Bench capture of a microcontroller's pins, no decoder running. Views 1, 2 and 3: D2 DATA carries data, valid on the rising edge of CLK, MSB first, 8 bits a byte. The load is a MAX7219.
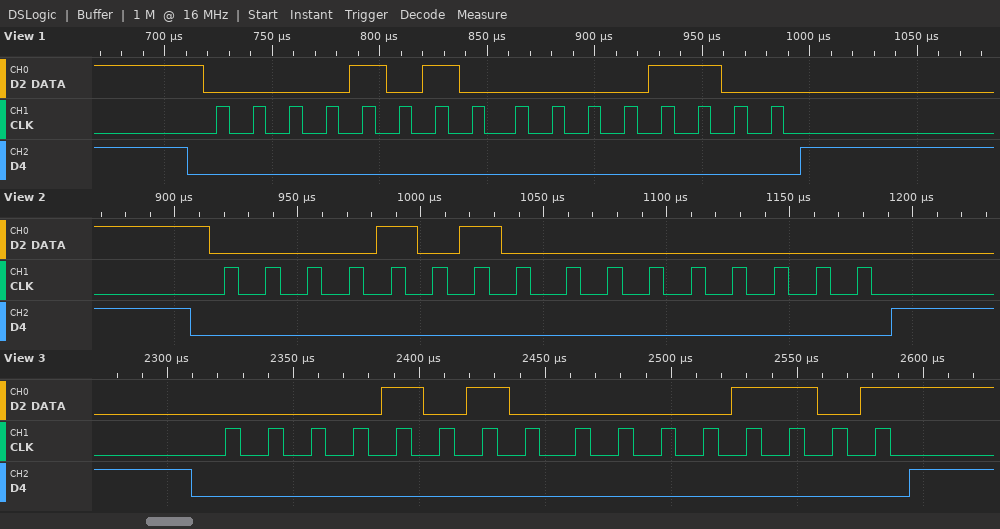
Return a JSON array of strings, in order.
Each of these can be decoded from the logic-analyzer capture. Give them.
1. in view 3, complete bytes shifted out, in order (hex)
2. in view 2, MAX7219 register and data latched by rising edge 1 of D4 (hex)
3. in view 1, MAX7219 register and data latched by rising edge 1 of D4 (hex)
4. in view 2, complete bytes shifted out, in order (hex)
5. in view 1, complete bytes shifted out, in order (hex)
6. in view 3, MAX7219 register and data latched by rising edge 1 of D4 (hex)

["0A 0D", "register 0xA, data 0x00", "register 0xA, data 0x0C", "0x0A 0x00", "0A 0C", "register 0xA, data 0x0D"]
